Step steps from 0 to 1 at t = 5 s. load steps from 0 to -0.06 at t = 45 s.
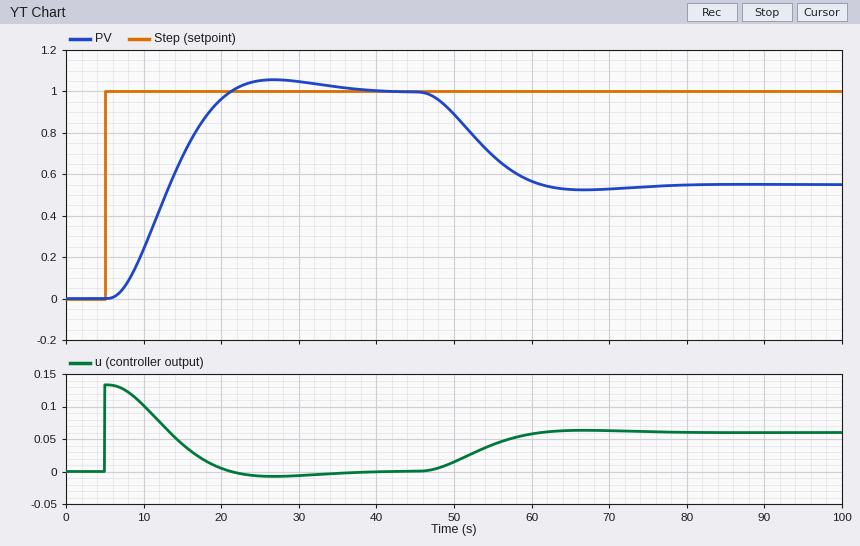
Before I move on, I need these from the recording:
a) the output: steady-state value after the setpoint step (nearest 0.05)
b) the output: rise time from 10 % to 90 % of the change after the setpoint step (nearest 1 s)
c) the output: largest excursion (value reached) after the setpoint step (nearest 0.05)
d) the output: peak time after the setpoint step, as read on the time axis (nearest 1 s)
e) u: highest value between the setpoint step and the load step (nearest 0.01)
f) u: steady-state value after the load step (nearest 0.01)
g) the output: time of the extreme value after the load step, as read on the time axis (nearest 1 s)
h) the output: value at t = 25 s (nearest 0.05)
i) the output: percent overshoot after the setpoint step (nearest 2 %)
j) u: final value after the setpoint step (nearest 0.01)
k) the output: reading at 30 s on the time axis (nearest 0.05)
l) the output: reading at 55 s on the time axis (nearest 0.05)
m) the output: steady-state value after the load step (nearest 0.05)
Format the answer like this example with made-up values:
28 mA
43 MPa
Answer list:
1.00
10 s
1.05
27 s
0.13
0.06
67 s
1.05
6 %
0.00
1.05
0.70
0.55
